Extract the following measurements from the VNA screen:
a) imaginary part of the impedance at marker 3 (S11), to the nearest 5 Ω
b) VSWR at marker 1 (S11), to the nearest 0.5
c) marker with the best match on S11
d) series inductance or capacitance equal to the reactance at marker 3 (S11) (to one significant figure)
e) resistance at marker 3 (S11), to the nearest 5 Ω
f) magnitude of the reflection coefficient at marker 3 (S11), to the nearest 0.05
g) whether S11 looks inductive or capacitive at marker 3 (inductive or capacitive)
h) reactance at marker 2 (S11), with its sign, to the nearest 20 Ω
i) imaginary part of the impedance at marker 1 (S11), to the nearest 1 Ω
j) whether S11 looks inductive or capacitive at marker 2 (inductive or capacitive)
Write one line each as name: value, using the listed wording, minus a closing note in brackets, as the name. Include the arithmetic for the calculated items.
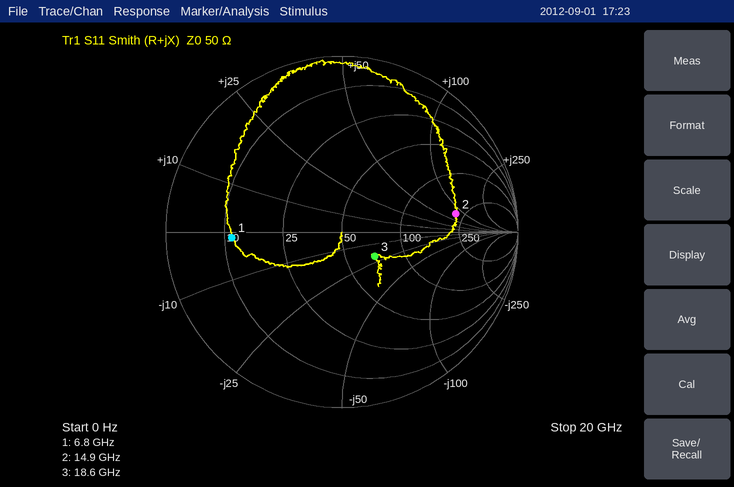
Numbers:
imaginary part of the impedance at marker 3 (S11), to the nearest 5 Ω: -20 Ω
VSWR at marker 1 (S11), to the nearest 0.5: 4.5
marker with the best match on S11: marker 3
series inductance or capacitance equal to the reactance at marker 3 (S11): C = 1/(2π × 18.6 GHz × 20 Ω) ≈ 428 fF, so 400 fF to one significant figure
resistance at marker 3 (S11), to the nearest 5 Ω: 70 Ω
magnitude of the reflection coefficient at marker 3 (S11), to the nearest 0.05: 0.25
whether S11 looks inductive or capacitive at marker 3: capacitive
reactance at marker 2 (S11), with its sign, to the nearest 20 Ω: +80 Ω
imaginary part of the impedance at marker 1 (S11), to the nearest 1 Ω: -1 Ω
whether S11 looks inductive or capacitive at marker 2: inductive
